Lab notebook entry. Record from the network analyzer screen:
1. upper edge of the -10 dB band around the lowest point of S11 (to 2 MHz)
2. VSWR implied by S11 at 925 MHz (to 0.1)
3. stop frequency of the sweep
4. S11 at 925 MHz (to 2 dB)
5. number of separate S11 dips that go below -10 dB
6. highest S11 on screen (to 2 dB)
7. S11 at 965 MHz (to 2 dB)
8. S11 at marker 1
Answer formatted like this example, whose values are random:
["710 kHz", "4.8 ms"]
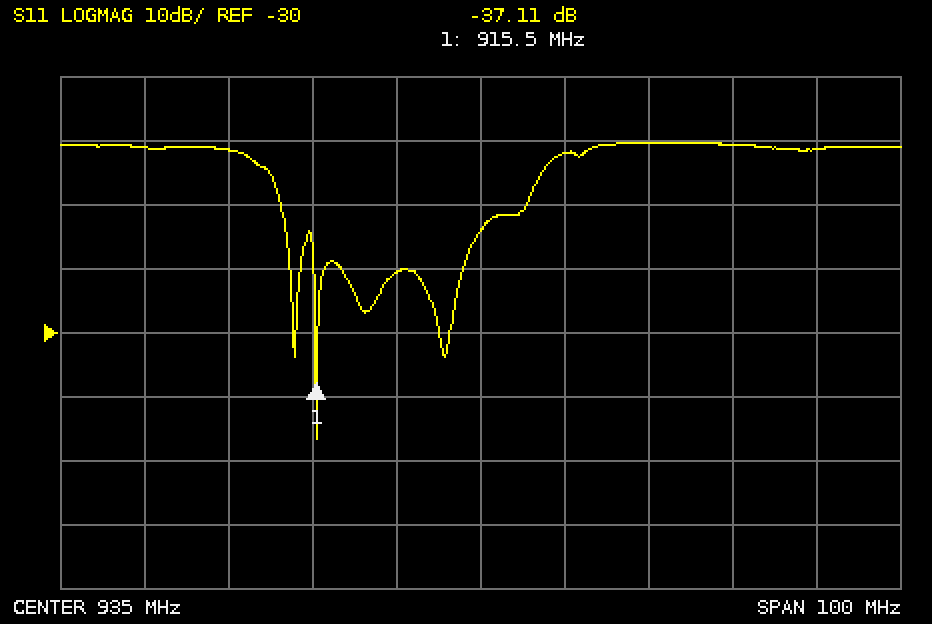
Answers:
["940 MHz", "1.2", "985 MHz", "-20 dB", "4", "0 dB", "0 dB", "-37.11 dB"]
